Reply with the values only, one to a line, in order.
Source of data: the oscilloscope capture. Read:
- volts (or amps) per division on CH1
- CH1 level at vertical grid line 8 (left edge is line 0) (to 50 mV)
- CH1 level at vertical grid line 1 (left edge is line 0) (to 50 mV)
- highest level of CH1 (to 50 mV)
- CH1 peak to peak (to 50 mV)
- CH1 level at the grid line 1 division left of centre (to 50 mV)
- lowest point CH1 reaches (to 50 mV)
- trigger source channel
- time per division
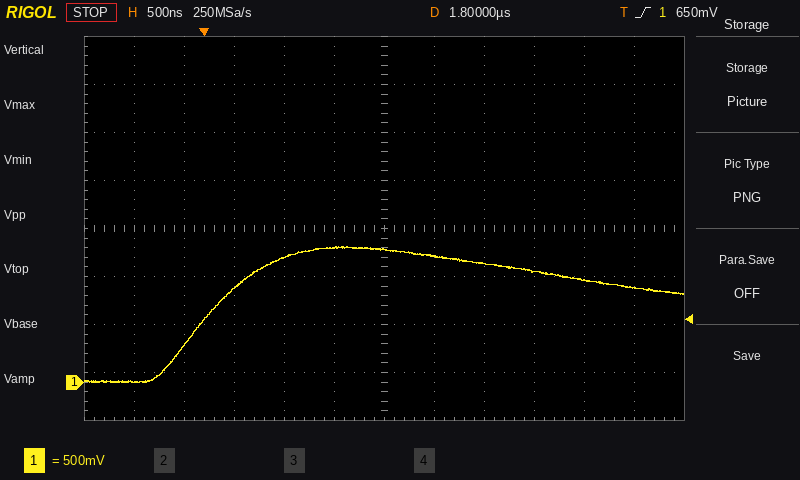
500 mV
1.25 V
0 mV
1.40 V
1.40 V
1.40 V
0 mV
CH1
500 ns
